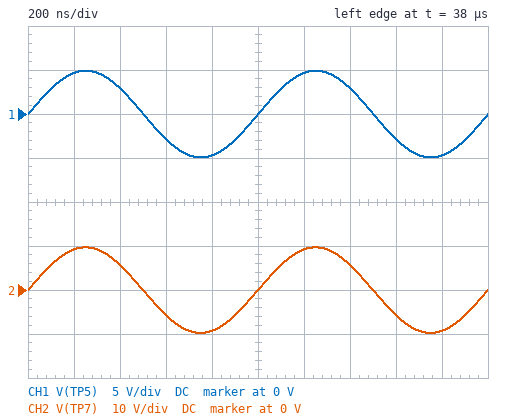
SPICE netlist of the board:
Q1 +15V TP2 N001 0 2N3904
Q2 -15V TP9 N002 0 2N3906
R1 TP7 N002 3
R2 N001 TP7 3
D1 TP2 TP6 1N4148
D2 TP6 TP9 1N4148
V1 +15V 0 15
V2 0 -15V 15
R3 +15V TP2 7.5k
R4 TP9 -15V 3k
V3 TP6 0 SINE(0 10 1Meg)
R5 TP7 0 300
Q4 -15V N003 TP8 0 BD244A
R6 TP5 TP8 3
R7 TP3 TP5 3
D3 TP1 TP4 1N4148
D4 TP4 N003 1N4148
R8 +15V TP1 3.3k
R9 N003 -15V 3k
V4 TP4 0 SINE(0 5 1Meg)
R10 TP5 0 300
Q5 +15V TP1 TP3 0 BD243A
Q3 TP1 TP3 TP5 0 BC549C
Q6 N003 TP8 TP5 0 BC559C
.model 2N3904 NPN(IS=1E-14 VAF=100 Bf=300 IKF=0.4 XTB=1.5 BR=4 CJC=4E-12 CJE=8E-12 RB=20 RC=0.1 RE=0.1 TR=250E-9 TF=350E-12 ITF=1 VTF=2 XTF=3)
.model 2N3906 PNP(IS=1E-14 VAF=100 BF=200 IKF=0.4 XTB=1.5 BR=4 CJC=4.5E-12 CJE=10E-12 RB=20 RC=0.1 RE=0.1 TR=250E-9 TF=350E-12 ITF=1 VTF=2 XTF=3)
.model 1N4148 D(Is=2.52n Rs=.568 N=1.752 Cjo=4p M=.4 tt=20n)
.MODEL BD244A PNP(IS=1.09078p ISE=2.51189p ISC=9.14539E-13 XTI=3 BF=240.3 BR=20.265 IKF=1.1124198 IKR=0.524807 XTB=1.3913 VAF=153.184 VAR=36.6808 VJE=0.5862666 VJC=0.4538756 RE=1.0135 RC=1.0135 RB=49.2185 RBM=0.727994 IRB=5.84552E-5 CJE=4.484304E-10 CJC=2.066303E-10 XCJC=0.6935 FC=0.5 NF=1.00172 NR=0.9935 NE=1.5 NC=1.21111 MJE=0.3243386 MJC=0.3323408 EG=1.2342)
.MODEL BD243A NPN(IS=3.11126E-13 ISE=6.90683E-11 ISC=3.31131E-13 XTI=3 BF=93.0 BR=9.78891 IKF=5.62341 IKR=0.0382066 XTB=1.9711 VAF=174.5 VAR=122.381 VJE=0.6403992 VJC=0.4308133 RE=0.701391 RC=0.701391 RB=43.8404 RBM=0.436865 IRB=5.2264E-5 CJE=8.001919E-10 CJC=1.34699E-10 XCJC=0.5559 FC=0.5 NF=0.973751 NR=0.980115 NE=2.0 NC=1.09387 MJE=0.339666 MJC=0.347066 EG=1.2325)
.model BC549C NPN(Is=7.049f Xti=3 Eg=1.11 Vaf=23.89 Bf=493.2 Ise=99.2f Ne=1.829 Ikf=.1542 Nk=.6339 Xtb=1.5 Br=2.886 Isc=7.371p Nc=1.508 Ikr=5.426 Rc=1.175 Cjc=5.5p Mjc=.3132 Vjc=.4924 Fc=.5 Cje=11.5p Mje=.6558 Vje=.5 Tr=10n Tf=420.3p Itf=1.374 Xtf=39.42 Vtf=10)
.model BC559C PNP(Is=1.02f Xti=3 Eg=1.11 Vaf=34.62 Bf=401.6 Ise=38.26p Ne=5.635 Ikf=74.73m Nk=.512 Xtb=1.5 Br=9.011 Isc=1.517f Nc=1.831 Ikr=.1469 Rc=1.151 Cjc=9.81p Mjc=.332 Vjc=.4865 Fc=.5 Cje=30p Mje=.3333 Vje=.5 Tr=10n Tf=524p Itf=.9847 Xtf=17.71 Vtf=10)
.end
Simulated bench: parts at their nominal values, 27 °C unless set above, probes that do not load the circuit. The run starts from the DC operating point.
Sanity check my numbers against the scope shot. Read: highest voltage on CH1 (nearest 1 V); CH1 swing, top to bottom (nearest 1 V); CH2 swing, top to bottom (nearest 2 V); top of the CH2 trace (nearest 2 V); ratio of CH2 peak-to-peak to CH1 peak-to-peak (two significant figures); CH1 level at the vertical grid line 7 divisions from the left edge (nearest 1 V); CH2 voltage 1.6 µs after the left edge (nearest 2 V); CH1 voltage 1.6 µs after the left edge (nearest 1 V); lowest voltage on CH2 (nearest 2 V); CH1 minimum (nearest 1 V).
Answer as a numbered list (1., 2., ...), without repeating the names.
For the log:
1. 5 V
2. 10 V
3. 20 V
4. 10 V
5. 2.0
6. 3 V
7. -6 V
8. -3 V
9. -10 V
10. -5 V
